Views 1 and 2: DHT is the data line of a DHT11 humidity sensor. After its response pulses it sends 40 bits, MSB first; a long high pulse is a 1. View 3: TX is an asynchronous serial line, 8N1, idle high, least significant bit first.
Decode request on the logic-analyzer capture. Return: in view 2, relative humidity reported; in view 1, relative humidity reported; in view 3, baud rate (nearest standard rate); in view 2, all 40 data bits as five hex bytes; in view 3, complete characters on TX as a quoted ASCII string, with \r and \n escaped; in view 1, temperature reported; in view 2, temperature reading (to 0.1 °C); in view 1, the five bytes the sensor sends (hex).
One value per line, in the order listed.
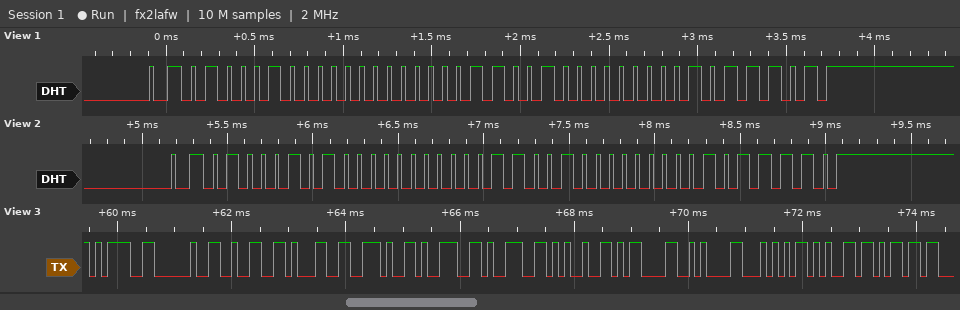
69 %
68 %
9600 baud
45 00 19 00 5E
"= 21.99%\r\nTem"
25.0 °C
25.0 °C
44 00 19 00 5D
